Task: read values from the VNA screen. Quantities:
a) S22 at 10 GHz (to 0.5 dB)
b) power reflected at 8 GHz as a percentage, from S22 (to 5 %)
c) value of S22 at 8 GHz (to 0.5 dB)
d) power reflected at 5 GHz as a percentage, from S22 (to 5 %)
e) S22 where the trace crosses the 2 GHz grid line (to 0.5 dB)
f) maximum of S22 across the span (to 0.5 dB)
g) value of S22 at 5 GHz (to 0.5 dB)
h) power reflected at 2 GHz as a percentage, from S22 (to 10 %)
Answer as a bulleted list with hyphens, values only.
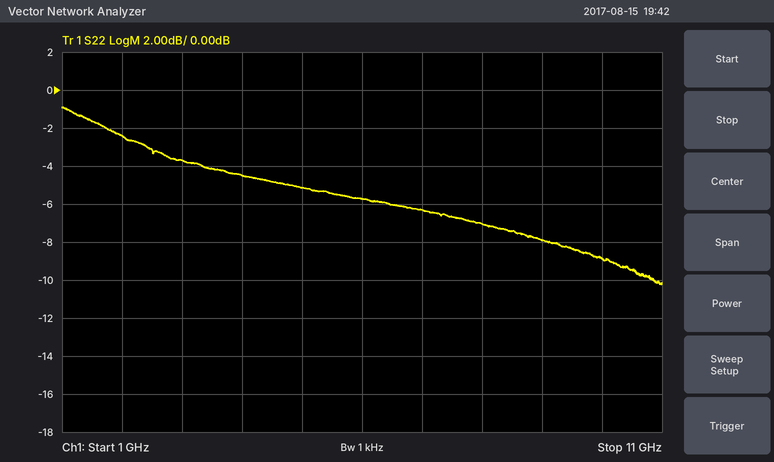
- -9.0 dB
- 20 %
- -7.0 dB
- 30 %
- -2.5 dB
- -1.0 dB
- -5.0 dB
- 60 %
